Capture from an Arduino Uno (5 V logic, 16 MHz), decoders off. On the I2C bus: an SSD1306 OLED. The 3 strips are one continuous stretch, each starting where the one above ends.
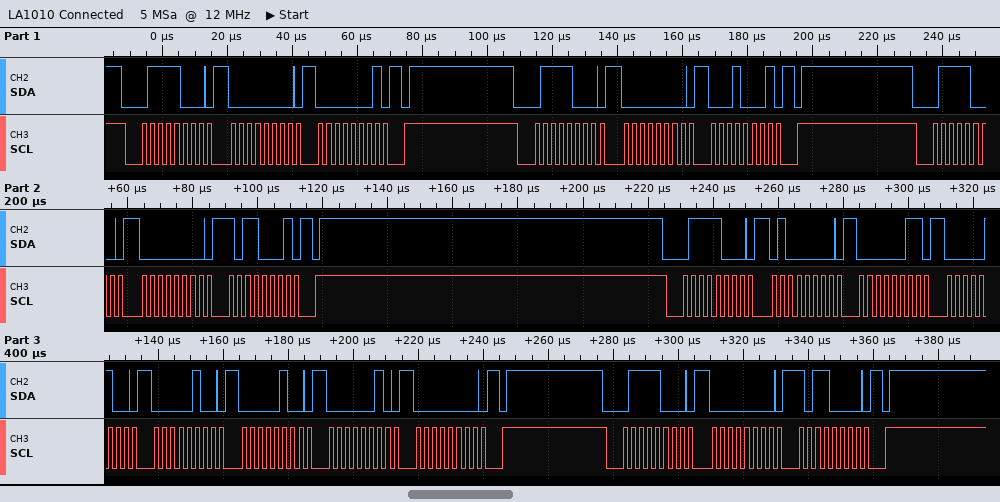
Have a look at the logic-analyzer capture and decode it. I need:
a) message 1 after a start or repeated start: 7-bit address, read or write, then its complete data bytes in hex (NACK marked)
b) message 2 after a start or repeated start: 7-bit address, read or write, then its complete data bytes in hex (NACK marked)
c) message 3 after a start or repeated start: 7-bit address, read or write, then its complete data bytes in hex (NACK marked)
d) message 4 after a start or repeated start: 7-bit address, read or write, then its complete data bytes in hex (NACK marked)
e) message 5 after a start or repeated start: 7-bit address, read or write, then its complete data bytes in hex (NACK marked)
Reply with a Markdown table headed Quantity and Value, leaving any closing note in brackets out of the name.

| Quantity | Value |
|---|---|
| message 1 after a start or repeated start: 7-bit address, read or write, then its complete data bytes in hex | 0x3C write: 00 01 |
| message 2 after a start or repeated start: 7-bit address, read or write, then its complete data bytes in hex | 0x3C write: 00 11 |
| message 3 after a start or repeated start: 7-bit address, read or write, then its complete data bytes in hex | 0x3C write: 00 B1 |
| message 4 after a start or repeated start: 7-bit address, read or write, then its complete data bytes in hex | 0x3C write: 40 03 04 04 04 02 00 |
| message 5 after a start or repeated start: 7-bit address, read or write, then its complete data bytes in hex | 0x3C write: 00 B0 |
